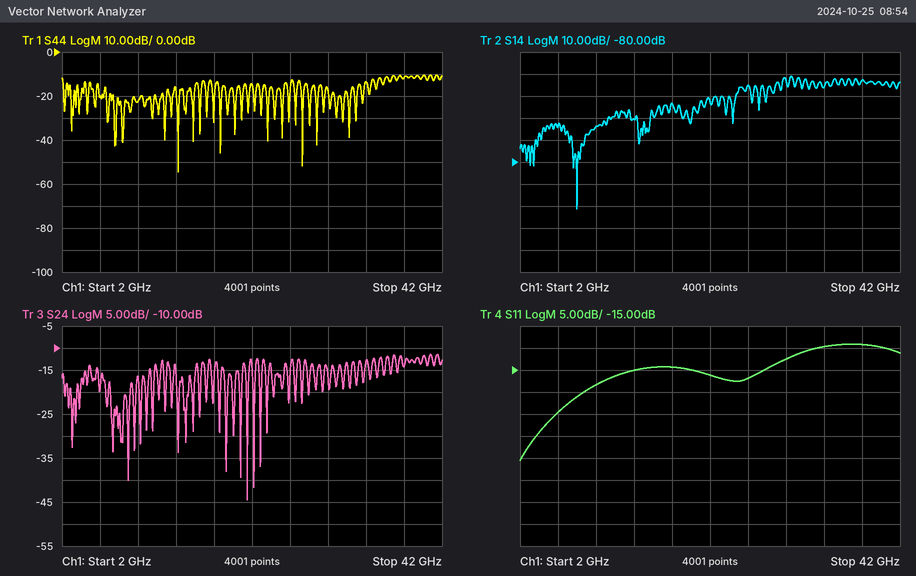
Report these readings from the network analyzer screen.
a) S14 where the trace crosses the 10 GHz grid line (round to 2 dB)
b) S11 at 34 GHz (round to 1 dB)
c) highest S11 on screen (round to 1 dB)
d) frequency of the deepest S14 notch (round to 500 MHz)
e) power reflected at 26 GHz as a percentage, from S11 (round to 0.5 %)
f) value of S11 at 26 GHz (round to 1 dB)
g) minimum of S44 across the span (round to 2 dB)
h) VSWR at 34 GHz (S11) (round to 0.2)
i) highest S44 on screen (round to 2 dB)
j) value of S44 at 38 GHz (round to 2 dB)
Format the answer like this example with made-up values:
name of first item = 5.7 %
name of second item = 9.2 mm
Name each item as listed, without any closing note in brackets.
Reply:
S14 where the trace crosses the 10 GHz grid line = -64 dB
S11 at 34 GHz = -10 dB
highest S11 on screen = -9 dB
frequency of the deepest S14 notch = 8.0 GHz
power reflected at 26 GHz as a percentage, from S11 = 2.0 %
value of S11 at 26 GHz = -17 dB
minimum of S44 across the span = -54 dB
VSWR at 34 GHz (S11) = 2.0
highest S44 on screen = -10 dB
value of S44 at 38 GHz = -12 dB
